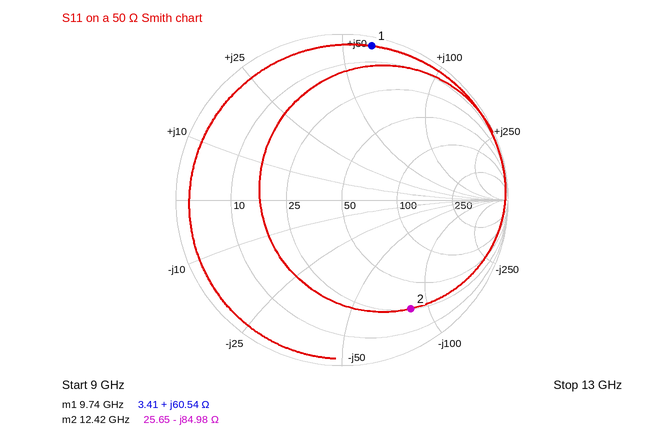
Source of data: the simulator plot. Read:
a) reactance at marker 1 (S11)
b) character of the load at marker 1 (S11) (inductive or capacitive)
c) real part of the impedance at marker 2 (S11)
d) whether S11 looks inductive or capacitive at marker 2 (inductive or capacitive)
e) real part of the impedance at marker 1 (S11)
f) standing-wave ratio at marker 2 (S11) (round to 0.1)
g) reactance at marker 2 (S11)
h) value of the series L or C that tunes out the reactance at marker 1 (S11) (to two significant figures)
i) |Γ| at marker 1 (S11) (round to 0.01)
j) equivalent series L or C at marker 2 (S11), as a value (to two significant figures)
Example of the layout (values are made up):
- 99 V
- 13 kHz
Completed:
- +60.54 Ω
- inductive
- 25.65 Ω
- capacitive
- 3.41 Ω
- 8.0
- -84.98 Ω
- 270 fF
- 0.95
- 150 fF
